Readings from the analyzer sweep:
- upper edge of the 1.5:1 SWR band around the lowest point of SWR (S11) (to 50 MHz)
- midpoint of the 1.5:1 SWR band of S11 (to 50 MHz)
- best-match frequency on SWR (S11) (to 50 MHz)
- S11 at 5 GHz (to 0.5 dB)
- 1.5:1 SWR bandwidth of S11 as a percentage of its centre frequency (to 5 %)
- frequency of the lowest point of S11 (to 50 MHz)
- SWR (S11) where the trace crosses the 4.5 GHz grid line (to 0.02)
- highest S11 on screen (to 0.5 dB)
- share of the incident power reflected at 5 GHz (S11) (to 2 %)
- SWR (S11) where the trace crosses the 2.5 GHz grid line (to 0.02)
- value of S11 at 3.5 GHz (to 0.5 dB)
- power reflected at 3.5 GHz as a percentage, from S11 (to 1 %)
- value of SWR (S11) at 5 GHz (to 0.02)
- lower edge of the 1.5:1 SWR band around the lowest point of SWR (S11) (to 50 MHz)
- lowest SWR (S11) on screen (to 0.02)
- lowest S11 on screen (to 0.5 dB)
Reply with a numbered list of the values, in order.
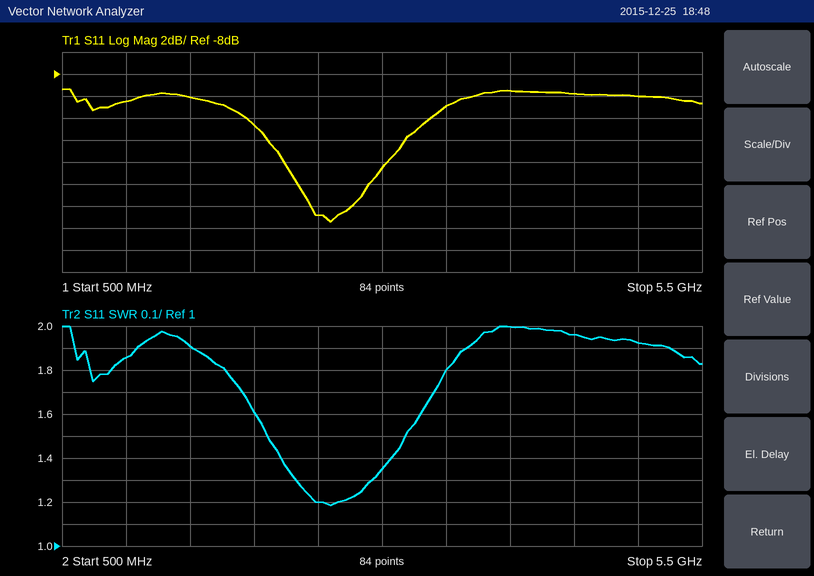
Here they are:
1. 3.20 GHz
2. 2.65 GHz
3. 2.60 GHz
4. -10.0 dB
5. 40 %
6. 2.60 GHz
7. 1.96
8. -9.5 dB
9. 10 %
10. 1.20
11. -11.0 dB
12. 8 %
13. 1.92
14. 2.10 GHz
15. 1.18
16. -21.5 dB
